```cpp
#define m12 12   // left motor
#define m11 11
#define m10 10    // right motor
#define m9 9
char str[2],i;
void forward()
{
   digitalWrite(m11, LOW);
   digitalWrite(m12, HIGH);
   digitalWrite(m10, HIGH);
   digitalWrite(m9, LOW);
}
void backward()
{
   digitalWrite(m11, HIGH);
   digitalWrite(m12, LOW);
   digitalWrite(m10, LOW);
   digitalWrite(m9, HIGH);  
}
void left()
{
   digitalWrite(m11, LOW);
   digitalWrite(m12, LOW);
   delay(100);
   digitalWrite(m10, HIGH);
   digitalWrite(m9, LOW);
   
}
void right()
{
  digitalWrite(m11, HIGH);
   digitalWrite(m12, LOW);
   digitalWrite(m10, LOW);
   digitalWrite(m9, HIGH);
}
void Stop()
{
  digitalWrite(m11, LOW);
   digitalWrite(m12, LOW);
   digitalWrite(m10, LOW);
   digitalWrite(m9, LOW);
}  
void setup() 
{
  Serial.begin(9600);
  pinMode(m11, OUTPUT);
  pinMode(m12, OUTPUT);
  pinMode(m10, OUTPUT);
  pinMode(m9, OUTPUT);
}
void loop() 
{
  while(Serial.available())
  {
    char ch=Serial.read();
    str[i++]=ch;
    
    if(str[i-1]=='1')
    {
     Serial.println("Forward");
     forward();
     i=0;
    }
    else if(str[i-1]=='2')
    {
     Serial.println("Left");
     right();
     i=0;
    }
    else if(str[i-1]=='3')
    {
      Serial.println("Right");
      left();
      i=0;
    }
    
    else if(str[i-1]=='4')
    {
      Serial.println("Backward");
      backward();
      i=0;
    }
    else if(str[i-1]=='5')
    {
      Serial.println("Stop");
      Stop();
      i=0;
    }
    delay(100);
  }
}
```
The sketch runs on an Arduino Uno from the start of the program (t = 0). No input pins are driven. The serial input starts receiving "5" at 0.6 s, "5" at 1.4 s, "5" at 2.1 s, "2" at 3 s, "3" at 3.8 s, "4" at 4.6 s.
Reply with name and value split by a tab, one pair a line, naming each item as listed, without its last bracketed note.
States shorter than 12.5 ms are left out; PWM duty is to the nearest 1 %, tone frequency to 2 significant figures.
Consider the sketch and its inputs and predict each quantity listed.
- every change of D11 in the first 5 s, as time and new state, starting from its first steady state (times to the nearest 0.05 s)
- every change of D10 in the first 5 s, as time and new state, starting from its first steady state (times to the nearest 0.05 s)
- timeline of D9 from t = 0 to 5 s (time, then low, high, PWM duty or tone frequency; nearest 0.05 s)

every change of D11 in the first 5 s, as time and new state, starting from its first steady state	0 s low; 3 s high; 3.8 s low; 4.6 s high
every change of D10 in the first 5 s, as time and new state, starting from its first steady state	0 s low; 3.9 s high; 4.6 s low
timeline of D9 from t = 0 to 5 s	0 s low; 3 s high; 3.9 s low; 4.6 s high
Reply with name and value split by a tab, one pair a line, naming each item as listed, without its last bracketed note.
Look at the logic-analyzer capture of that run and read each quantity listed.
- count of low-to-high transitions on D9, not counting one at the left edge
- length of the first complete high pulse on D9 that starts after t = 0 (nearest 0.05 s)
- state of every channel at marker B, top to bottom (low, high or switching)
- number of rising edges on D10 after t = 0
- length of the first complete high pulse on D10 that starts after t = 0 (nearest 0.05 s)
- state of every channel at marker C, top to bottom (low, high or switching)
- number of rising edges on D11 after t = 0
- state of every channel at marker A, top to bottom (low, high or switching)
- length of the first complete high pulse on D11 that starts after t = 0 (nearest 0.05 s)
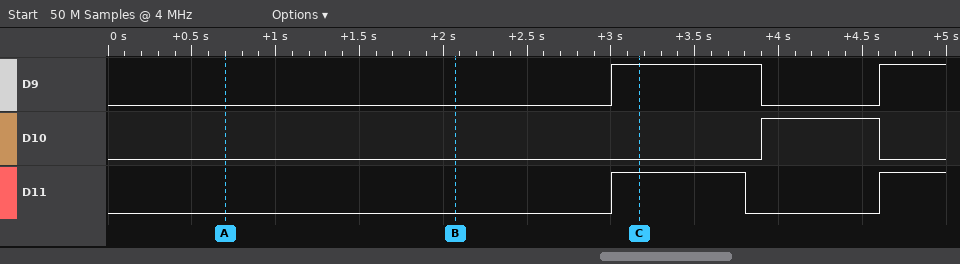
count of low-to-high transitions on D9, not counting one at the left edge	2
length of the first complete high pulse on D9 that starts after t = 0	0.90 s
state of every channel at marker B, top to bottom	D9 low, D10 low, D11 low
number of rising edges on D10 after t = 0	1
length of the first complete high pulse on D10 that starts after t = 0	0.70 s
state of every channel at marker C, top to bottom	D9 high, D10 low, D11 high
number of rising edges on D11 after t = 0	2
state of every channel at marker A, top to bottom	D9 low, D10 low, D11 low
length of the first complete high pulse on D11 that starts after t = 0	0.80 s
